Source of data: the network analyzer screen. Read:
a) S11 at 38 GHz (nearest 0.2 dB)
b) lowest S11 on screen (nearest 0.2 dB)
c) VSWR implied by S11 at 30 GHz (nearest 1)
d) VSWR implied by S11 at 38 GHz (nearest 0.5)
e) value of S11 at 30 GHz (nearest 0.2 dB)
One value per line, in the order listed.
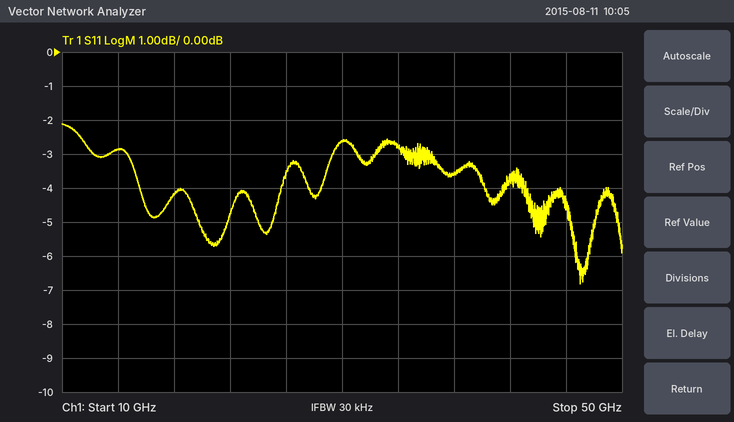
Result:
-3.6 dB
-6.8 dB
7
5.0
-2.6 dB
